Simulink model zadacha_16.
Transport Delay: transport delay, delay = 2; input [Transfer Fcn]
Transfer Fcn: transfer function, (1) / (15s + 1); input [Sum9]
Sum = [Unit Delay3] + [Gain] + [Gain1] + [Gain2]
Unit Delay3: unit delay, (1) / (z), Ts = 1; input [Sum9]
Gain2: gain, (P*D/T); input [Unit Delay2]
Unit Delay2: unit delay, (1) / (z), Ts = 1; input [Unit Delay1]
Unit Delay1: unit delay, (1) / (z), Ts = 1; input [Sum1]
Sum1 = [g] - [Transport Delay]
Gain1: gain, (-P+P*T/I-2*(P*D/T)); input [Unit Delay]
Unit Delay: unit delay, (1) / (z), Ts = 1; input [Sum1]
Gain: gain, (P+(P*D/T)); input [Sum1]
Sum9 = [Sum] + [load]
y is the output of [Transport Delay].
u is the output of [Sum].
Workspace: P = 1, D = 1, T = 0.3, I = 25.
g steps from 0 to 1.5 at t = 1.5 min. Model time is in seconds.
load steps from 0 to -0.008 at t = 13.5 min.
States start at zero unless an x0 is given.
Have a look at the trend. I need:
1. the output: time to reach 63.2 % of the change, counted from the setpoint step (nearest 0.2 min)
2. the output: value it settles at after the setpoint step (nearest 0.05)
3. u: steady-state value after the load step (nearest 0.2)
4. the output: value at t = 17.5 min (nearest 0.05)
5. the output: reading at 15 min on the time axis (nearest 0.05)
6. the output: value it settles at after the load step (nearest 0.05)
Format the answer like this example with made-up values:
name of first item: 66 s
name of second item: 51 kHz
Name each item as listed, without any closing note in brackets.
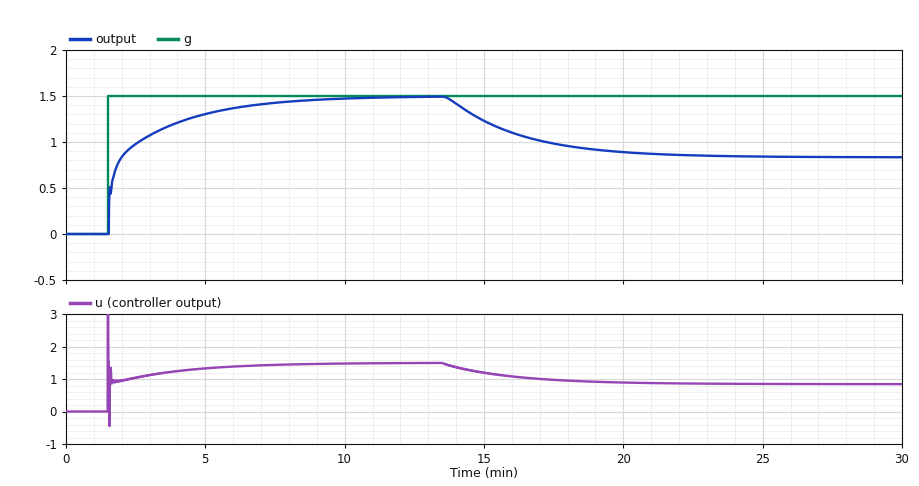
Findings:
the output: time to reach 63.2 % of the change, counted from the setpoint step: 0.8 min
the output: value it settles at after the setpoint step: 1.50
u: steady-state value after the load step: 0.8
the output: value at t = 17.5 min: 1.00
the output: reading at 15 min on the time axis: 1.25
the output: value it settles at after the load step: 0.85
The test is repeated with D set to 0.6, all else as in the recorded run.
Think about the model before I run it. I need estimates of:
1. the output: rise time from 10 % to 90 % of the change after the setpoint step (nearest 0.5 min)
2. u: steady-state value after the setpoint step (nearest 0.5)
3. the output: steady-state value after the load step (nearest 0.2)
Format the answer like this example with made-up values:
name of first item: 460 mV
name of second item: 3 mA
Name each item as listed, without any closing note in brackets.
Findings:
the output: rise time from 10 % to 90 % of the change after the setpoint step: 4.0 min
u: steady-state value after the setpoint step: 1.5
the output: steady-state value after the load step: 0.8
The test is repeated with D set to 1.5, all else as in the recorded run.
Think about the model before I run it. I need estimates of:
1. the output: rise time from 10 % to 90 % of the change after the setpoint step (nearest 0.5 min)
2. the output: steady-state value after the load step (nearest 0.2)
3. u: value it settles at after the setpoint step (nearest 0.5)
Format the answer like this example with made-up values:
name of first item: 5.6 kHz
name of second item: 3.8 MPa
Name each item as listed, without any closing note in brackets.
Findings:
the output: rise time from 10 % to 90 % of the change after the setpoint step: 4.0 min
the output: steady-state value after the load step: 0.8
u: value it settles at after the setpoint step: 1.5
